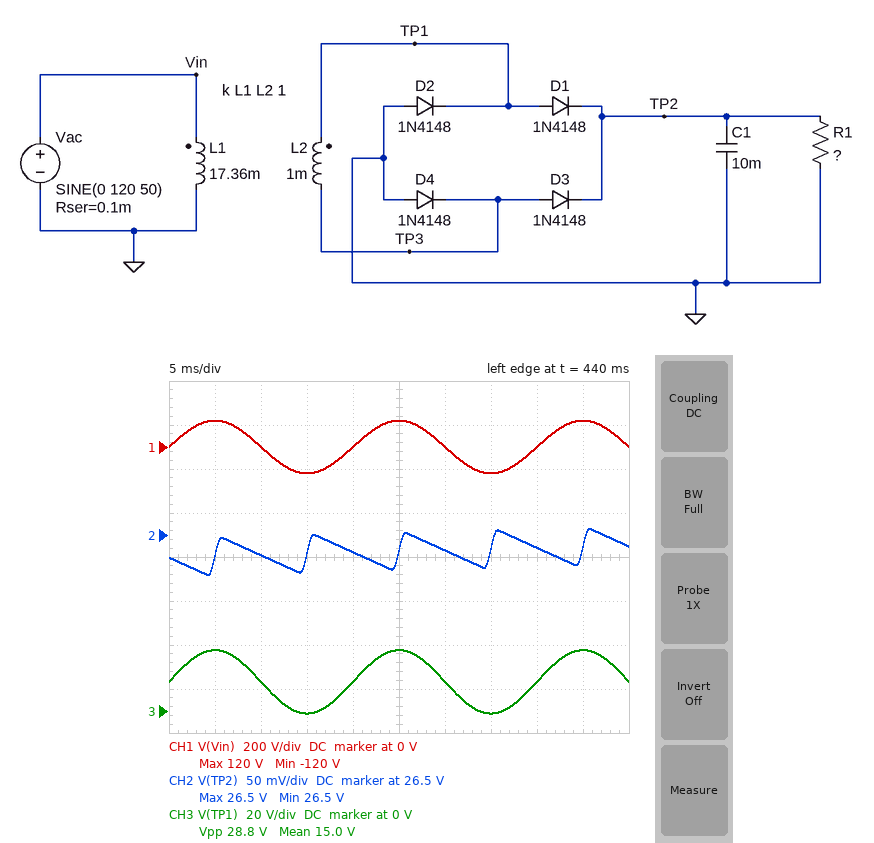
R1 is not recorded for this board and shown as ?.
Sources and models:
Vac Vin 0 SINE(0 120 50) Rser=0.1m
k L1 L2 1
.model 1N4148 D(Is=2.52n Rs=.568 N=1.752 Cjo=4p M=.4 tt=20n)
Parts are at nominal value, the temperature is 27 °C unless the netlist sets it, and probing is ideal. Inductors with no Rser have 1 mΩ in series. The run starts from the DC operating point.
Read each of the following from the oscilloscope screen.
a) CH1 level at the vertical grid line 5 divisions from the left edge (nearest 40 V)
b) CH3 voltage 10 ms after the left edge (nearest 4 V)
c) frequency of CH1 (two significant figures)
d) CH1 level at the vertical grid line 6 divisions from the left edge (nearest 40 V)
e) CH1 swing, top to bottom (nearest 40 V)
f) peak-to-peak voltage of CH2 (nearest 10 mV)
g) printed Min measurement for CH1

120 V
12 V
50 Hz
0 V
240 V
50 mV
-120 V
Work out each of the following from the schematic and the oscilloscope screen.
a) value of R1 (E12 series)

560 Ω
